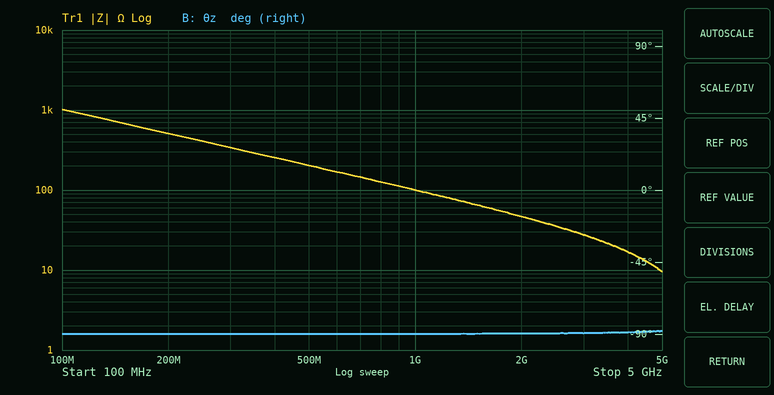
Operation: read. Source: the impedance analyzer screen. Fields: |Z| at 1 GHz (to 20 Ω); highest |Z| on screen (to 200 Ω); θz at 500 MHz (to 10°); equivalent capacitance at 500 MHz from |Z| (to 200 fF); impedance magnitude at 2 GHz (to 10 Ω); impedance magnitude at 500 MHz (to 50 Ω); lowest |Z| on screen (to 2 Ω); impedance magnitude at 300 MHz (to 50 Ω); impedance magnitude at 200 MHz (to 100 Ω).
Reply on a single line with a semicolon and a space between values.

100 Ω; 1.0 kΩ; -90°; 1.6 pF; 50 Ω; 200 Ω; 10 Ω; 350 Ω; 500 Ω
